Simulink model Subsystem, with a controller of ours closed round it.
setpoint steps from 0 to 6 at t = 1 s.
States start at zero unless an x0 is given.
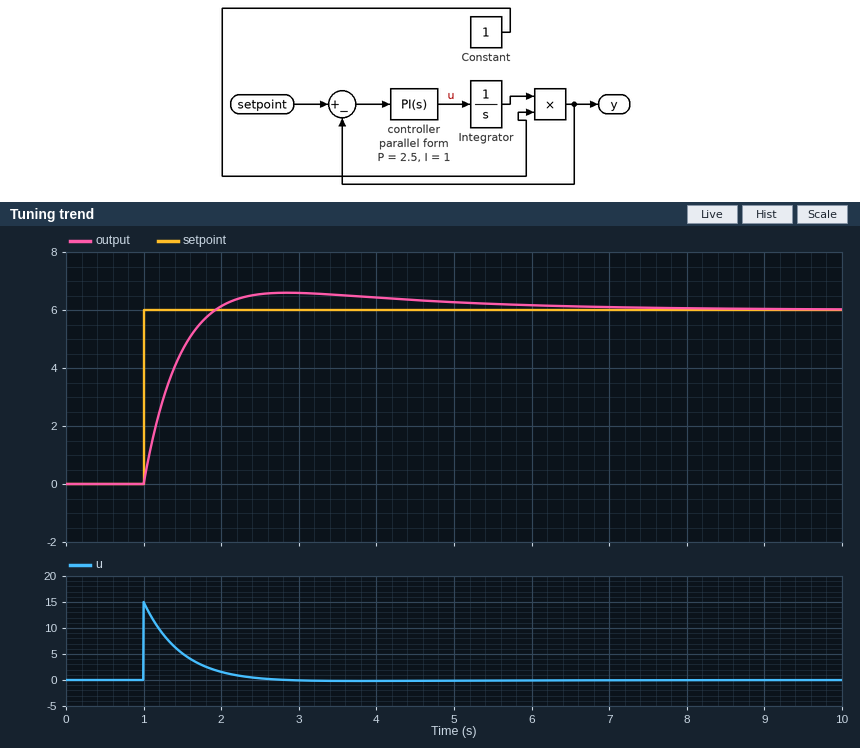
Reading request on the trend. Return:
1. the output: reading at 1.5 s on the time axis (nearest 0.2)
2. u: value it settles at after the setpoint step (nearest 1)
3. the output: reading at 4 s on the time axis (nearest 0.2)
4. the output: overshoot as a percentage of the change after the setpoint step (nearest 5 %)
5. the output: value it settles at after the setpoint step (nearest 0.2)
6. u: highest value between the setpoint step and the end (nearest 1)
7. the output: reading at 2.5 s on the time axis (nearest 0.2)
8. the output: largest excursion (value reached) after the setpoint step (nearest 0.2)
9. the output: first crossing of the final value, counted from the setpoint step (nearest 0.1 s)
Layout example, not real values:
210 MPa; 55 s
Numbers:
4.6; 0; 6.4; 10 %; 6.0; 15; 6.6; 6.6; 0.9 s
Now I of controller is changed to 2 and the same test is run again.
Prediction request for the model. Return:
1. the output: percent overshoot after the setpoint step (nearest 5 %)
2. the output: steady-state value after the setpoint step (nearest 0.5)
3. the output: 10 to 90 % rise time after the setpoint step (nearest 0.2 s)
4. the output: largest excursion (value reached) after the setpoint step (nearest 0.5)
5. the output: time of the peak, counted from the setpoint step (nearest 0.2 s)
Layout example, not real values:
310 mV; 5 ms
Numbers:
15 %; 6.0; 0.6 s; 7.0; 1.4 s
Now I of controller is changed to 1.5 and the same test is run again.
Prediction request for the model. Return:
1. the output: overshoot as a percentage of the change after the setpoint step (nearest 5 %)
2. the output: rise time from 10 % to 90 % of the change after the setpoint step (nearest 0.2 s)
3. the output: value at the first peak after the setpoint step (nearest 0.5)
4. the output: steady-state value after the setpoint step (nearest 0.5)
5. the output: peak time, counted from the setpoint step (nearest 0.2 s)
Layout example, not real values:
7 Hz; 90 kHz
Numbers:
15 %; 0.6 s; 7.0; 6.0; 1.6 s
